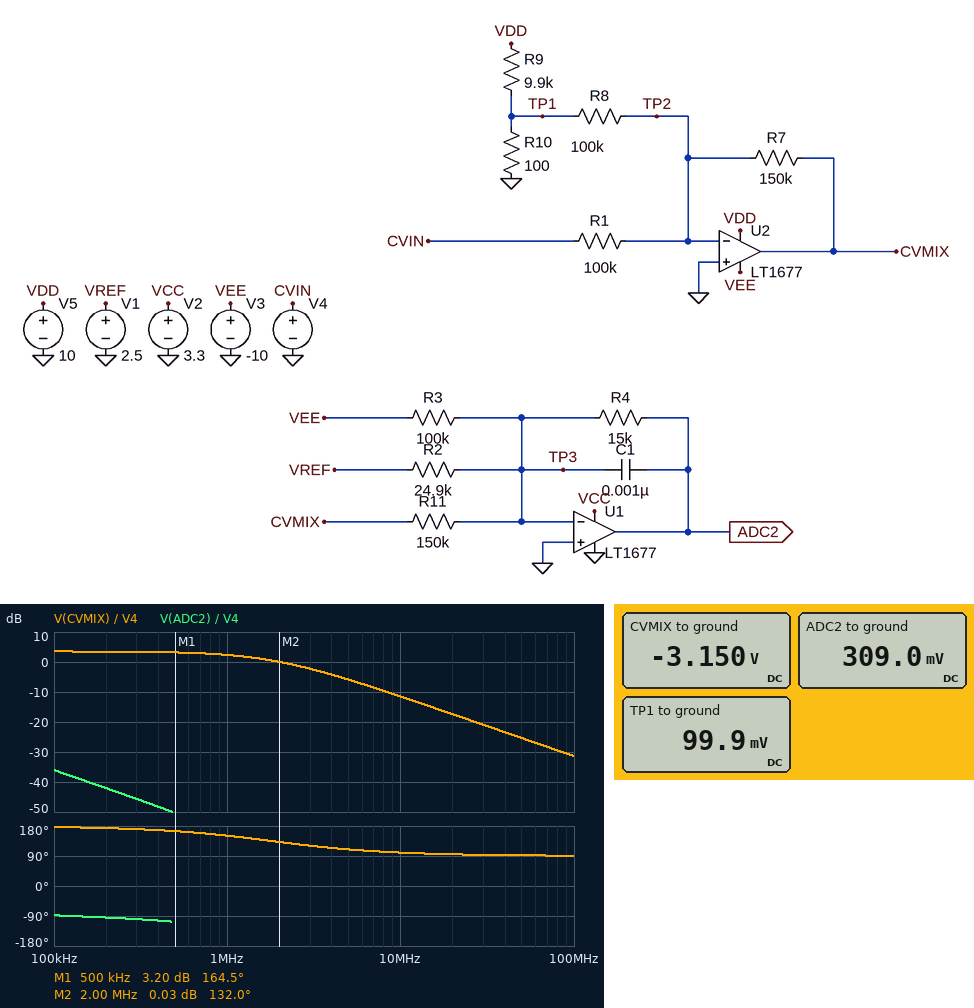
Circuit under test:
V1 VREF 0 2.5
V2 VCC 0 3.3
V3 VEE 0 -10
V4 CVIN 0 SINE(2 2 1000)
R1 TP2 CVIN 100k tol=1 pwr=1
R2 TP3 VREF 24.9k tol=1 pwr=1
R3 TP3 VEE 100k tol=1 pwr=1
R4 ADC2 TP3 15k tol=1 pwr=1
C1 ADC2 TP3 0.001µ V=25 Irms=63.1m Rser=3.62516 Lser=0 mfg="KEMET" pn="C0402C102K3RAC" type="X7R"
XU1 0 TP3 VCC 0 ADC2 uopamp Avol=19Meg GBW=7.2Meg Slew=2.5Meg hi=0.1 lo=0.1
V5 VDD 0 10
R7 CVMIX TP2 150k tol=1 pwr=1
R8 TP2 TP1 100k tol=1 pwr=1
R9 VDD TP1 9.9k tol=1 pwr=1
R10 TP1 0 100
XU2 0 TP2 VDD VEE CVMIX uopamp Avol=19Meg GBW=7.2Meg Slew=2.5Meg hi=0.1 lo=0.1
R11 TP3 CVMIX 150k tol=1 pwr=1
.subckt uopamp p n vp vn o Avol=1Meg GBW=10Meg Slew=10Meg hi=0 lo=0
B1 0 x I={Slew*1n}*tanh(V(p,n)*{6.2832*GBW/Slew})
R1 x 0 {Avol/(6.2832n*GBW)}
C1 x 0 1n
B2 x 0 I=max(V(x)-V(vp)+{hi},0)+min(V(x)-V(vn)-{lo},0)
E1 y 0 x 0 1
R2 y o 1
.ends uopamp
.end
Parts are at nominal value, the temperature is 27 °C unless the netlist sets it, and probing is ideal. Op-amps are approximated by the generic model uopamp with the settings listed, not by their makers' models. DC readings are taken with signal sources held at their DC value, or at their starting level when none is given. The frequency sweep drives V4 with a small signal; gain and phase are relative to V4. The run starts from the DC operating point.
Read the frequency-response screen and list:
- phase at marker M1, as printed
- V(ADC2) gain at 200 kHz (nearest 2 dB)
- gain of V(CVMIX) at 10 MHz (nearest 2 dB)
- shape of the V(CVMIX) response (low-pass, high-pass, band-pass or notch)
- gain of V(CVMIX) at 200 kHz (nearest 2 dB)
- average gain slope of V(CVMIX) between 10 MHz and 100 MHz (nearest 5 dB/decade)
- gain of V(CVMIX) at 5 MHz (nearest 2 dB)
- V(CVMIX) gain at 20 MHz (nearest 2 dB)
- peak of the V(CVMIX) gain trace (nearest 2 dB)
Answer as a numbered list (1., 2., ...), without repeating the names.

1. 164.5 deg
2. -42 dB
3. -12 dB
4. low-pass
5. 4 dB
6. -20 dB/decade
7. -6 dB
8. -18 dB
9. 4 dB
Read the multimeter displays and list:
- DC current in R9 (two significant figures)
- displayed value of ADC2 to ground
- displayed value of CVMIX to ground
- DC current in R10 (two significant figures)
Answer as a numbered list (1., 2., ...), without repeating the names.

1. 1.0 mA
2. 309.0 mV
3. -3.150 V
4. 1.0 mA
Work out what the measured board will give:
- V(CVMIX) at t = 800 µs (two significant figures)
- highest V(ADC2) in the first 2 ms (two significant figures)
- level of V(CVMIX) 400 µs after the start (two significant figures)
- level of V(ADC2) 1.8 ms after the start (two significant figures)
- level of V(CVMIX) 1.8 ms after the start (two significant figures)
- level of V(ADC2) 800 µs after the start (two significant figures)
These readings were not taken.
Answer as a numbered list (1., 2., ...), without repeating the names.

1. -300 mV
2. 610 mV
3. -4.9 V
4. 98 mV
5. -300 mV
6. 98 mV
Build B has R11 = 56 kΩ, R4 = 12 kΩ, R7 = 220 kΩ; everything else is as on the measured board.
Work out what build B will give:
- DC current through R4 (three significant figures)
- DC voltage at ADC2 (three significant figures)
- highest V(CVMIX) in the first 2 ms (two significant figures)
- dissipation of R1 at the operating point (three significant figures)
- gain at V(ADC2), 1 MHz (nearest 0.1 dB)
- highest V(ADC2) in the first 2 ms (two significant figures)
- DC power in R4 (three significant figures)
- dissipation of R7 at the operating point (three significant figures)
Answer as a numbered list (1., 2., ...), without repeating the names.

1. 82.1 µA
2. 985 mV
3. -220 mV
4. 40.0 µW
5. -46.1 dB
6. 1.9 V
7. 80.9 µW
8. 97.0 µW
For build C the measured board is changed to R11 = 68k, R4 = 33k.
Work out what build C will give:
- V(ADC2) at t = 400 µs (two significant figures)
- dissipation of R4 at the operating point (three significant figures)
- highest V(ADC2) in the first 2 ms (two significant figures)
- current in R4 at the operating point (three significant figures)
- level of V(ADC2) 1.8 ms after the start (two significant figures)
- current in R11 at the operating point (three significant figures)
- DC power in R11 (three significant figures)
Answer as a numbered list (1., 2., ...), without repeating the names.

1. 2.6 V
2. 69.6 µW
3. 2.9 V
4. 45.9 µA
5. 100 mV
6. 46.3 µA
7. 146 µW
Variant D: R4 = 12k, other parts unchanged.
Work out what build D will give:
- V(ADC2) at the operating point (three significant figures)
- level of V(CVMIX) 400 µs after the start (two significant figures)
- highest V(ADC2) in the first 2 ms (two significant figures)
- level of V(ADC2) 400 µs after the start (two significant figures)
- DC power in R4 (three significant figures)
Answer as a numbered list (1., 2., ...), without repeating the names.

1. 247 mV
2. -4.9 V
3. 490 mV
4. 400 mV
5. 5.09 µW
